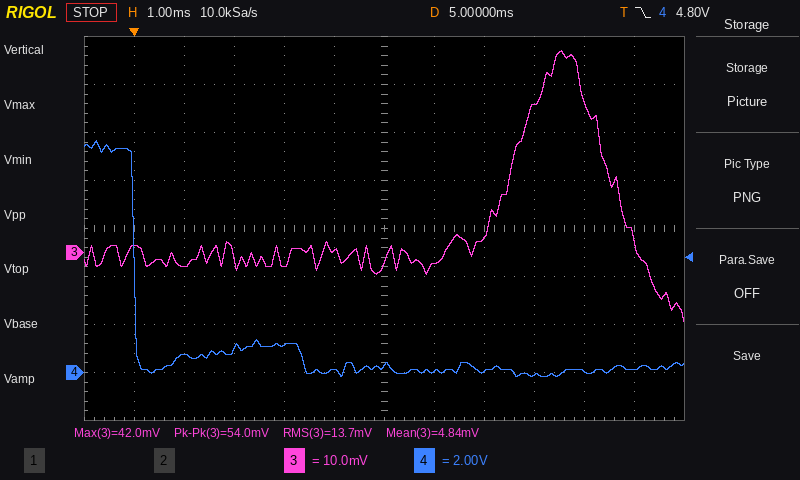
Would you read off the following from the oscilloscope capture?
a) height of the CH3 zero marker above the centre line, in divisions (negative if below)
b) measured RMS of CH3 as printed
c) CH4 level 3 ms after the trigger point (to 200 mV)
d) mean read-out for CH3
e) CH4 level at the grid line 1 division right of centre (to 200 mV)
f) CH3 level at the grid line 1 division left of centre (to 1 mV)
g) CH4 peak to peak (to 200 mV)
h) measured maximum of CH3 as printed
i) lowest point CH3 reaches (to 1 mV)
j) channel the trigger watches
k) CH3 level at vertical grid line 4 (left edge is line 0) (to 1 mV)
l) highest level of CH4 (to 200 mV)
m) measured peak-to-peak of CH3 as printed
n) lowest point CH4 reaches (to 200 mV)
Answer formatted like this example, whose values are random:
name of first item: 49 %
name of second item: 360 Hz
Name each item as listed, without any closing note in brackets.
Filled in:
height of the CH3 zero marker above the centre line, in divisions: -0.5 div
measured RMS of CH3 as printed: 13.7 mV
CH4 level 3 ms after the trigger point: 1.2 V
mean read-out for CH3: 4.84 mV
CH4 level at the grid line 1 division right of centre: 0.0 V
CH3 level at the grid line 1 division left of centre: 0 mV
CH4 peak to peak: 9.8 V
measured maximum of CH3 as printed: 42.0 mV
lowest point CH3 reaches: -14 mV
channel the trigger watches: CH4
CH3 level at vertical grid line 4 (left edge is line 0): -3 mV
highest level of CH4: 9.6 V
measured peak-to-peak of CH3 as printed: 54.0 mV
lowest point CH4 reaches: -200 mV
